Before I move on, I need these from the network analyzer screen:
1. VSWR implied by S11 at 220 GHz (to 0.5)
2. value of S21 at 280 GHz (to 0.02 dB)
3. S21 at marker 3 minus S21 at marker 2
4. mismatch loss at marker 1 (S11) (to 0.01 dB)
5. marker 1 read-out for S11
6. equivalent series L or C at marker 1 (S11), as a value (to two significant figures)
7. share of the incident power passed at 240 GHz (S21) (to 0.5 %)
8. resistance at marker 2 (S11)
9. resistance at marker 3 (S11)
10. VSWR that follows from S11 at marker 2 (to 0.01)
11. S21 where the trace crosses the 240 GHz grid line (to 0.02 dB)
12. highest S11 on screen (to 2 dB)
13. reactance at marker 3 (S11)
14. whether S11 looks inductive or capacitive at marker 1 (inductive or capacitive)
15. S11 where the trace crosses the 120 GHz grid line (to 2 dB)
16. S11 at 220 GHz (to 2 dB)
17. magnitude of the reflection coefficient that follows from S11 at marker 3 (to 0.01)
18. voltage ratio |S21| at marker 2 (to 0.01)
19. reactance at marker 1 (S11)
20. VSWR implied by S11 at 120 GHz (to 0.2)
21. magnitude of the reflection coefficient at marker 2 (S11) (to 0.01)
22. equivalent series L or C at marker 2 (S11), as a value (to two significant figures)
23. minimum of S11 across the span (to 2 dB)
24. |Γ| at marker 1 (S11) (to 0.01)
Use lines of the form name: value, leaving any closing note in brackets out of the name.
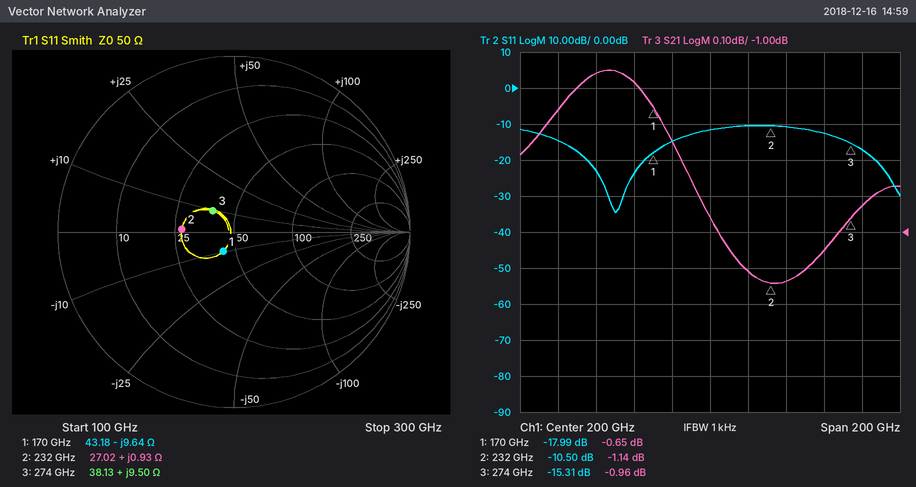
VSWR implied by S11 at 220 GHz: 2.0
value of S21 at 280 GHz: -0.92 dB
S21 at marker 3 minus S21 at marker 2: 0.18 dB
mismatch loss at marker 1 (S11): 0.07 dB
marker 1 read-out for S11: -17.99 dB
equivalent series L or C at marker 1 (S11), as a value: 97 fF
share of the incident power passed at 240 GHz (S21): 77.0 %
resistance at marker 2: 27.02 Ω
resistance at marker 3: 38.13 Ω
VSWR that follows from S11 at marker 2: 1.85
S21 where the trace crosses the 240 GHz grid line: -1.14 dB
highest S11 on screen: -10 dB
reactance at marker 3: +9.50 Ω
whether S11 looks inductive or capacitive at marker 1: capacitive
S11 where the trace crosses the 120 GHz grid line: -14 dB
S11 at 220 GHz: -10 dB
magnitude of the reflection coefficient that follows from S11 at marker 3: 0.17
voltage ratio |S21| at marker 2: 0.88
reactance at marker 1: -9.64 Ω
VSWR implied by S11 at 120 GHz: 1.4
magnitude of the reflection coefficient at marker 2 (S11): 0.30
equivalent series L or C at marker 2 (S11), as a value: 640 fH
minimum of S11 across the span: -34 dB
|Γ| at marker 1 (S11): 0.13
